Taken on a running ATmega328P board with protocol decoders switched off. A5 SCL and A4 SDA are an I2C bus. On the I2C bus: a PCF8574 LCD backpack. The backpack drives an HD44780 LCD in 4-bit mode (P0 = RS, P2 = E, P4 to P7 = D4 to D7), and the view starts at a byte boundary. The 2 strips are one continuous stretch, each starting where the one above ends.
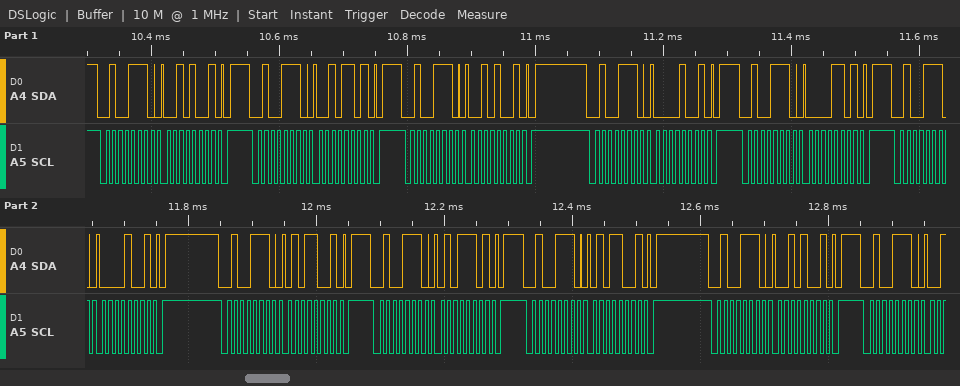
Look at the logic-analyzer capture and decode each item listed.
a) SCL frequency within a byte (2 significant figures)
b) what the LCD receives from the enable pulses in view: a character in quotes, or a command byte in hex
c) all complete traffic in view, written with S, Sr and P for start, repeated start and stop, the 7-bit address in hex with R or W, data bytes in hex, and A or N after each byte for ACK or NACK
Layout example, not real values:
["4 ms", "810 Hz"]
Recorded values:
["100 kHz", "' '", "S 27W A 29 A P S 27W A 2D A P S 27W A 29 A P S 27W A 09 A P S 27W A 0D A P S 27W A 09 A P S 27W A 59 A P S 27W A 5D A P S 27W A 59 A P S 27W A 29 A P S 27W A"]
